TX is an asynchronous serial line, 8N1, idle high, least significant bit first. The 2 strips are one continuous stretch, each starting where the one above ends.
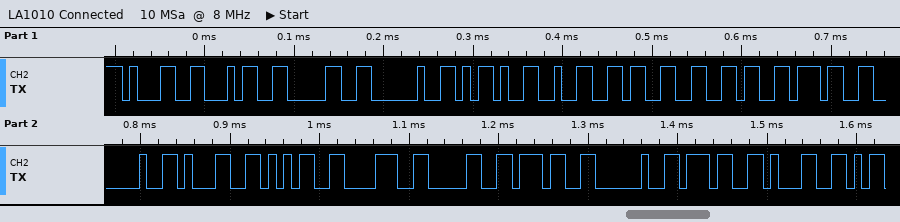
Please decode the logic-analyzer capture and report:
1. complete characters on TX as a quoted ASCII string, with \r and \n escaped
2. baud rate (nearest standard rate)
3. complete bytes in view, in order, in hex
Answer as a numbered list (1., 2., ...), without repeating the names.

1. "140 -2367 15807 71"
2. 115200 baud
3. 31 34 30 20 2D 32 33 36 37 20 31 35 38 30 37 20 37 31
